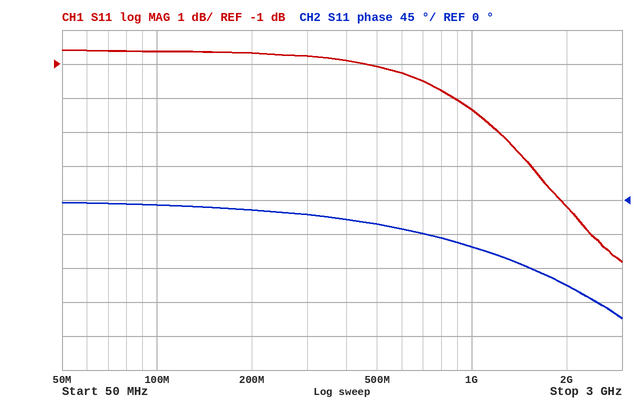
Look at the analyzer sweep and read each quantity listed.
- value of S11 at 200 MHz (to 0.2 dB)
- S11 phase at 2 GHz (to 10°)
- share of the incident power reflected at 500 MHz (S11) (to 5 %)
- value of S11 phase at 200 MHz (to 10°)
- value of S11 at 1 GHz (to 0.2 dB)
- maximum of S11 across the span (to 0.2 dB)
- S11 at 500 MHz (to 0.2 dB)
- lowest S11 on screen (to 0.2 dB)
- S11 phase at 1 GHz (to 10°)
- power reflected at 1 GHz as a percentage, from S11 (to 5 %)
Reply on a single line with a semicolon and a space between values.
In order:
-0.6 dB; -110°; 80 %; -10°; -2.4 dB; -0.6 dB; -1.0 dB; -6.8 dB; -60°; 60 %
